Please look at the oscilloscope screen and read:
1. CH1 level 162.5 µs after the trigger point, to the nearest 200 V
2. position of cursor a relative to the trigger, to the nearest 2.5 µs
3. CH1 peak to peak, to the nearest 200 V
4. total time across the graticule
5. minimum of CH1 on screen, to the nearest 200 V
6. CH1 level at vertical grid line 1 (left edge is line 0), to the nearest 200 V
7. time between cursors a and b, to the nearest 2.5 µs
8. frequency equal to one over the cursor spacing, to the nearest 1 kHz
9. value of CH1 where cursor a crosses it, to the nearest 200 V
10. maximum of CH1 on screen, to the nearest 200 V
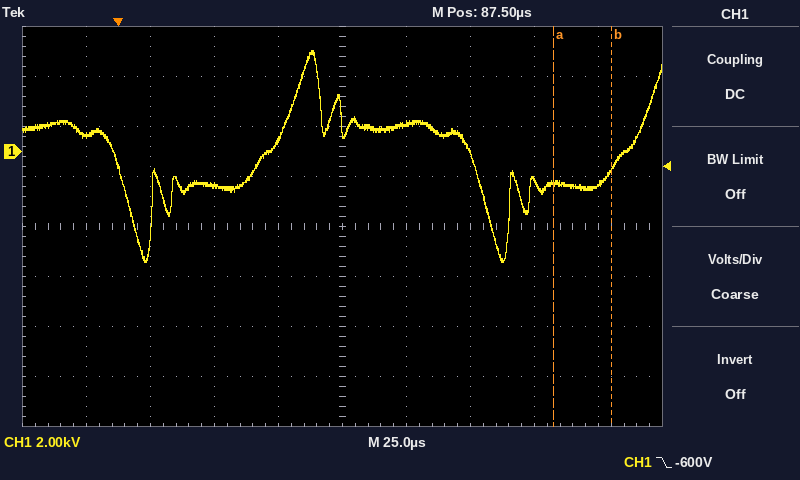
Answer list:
-1.2 kV
+170.0 µs
8.4 kV
250 µs
-4.4 kV
600 V
22.5 µs
44 kHz
-1.2 kV
4.0 kV
